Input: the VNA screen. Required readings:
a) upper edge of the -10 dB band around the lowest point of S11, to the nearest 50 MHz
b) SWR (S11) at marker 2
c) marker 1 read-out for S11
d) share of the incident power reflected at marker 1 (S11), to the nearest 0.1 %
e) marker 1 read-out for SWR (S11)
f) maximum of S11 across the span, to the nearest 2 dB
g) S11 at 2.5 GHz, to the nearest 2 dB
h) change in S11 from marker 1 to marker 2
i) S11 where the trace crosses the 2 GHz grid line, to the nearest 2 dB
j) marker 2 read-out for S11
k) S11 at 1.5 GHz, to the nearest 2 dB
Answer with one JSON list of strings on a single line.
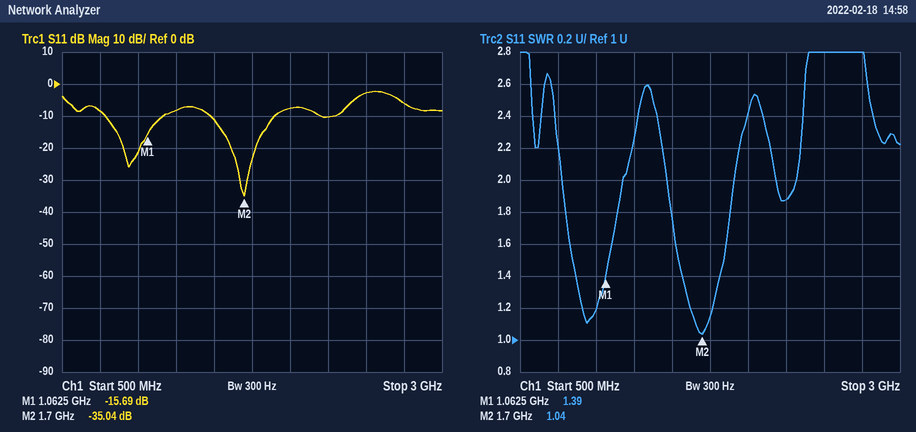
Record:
["1.90 GHz", "1.04", "-15.69 dB", "2.7 %", "1.39", "-2 dB", "-2 dB", "-19.35 dB", "-8 dB", "-35.04 dB", "-12 dB"]
